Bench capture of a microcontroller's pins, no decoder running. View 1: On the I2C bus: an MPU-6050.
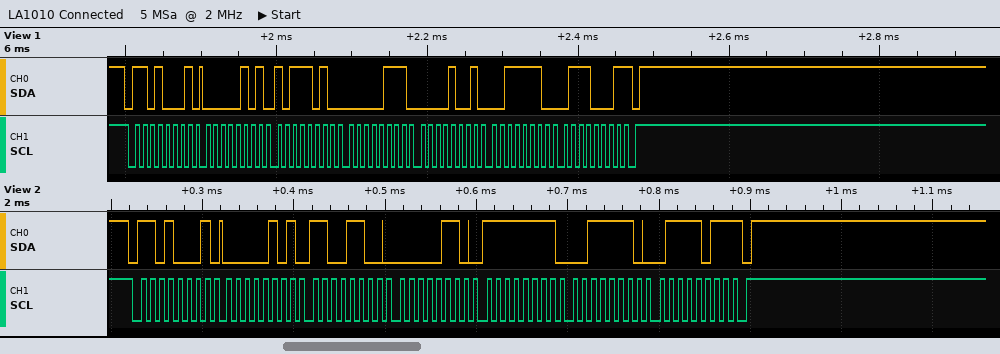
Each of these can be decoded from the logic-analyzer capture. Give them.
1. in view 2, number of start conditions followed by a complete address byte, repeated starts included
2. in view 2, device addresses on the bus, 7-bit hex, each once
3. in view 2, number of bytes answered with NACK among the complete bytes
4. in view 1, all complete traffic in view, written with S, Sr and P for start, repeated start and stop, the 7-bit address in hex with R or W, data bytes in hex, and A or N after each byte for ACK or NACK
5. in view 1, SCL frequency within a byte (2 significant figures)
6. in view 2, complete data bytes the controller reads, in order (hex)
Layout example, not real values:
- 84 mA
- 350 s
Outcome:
- 1
- 0x68
- 1
- S 68R A 05 A BA A 07 A 09 A 3E A 71 N P
- 100 kHz
- 05 CC 06 FF 3E 7B
